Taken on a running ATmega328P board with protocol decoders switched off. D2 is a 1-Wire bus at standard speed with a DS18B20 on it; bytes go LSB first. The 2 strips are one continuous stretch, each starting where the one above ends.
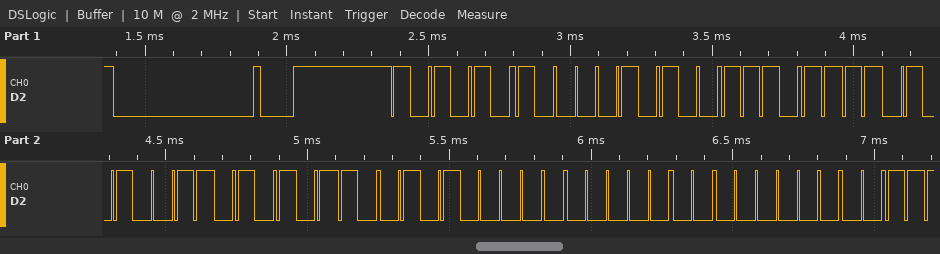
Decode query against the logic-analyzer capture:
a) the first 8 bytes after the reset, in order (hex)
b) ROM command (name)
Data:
55 28 F7 CA 6A 0A 00 00
Match ROM
